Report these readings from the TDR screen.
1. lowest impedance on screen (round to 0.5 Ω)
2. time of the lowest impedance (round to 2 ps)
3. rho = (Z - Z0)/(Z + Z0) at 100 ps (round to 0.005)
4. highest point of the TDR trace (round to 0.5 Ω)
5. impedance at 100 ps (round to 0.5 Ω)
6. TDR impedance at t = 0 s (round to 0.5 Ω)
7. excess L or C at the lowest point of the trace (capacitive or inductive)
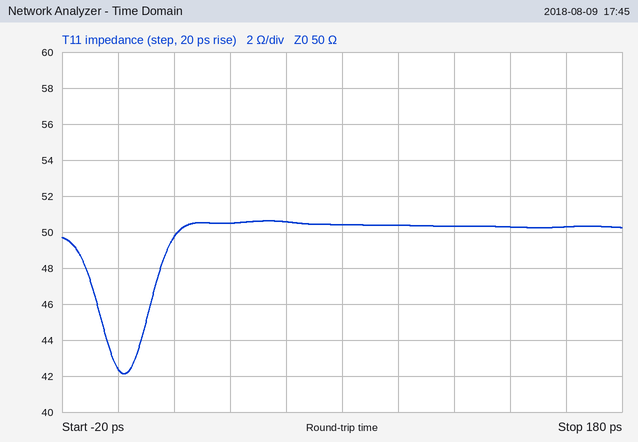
42.0 Ω
2 ps
+0.005
50.5 Ω
50.5 Ω
42.5 Ω
capacitive
